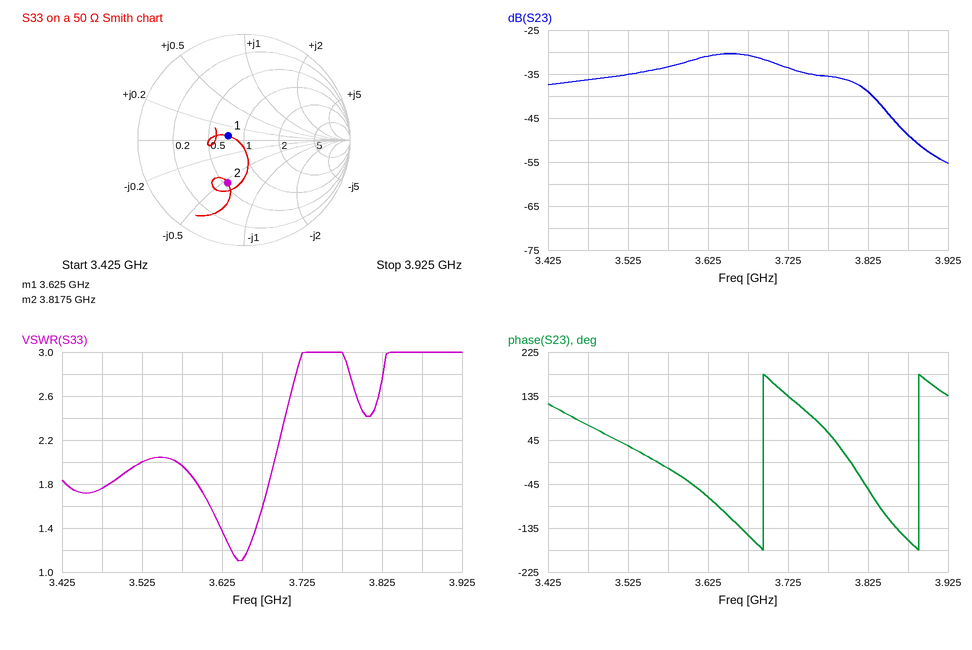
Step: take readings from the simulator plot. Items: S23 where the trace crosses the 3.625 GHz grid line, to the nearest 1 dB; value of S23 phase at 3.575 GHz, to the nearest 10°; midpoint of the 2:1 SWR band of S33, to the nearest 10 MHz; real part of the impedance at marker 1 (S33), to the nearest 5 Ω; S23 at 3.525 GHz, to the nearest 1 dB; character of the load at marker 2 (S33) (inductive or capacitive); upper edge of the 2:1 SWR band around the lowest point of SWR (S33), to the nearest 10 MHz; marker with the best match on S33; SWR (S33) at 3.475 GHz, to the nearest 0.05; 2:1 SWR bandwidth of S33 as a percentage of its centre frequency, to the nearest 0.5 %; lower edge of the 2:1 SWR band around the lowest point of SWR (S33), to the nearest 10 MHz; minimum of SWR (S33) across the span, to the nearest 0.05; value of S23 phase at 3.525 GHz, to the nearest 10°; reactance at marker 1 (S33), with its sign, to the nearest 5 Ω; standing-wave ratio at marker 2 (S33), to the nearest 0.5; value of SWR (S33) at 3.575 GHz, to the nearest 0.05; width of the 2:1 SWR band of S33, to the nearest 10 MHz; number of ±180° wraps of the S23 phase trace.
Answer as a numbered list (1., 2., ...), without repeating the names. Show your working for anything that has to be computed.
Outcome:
1. -31 dB
2. -10°
3. 3.63 GHz
4. 35 Ω
5. -35 dB
6. capacitive
7. 3.69 GHz
8. marker 1
9. 1.75
10. 120 MHz / 3.63 GHz ≈ 3.31 %, so 3.5 % to the nearest 0.5 %
11. 3.57 GHz
12. 1.10
13. 30°
14. +5 Ω
15. 2.5
16. 1.95
17. 3.69 GHz − 3.57 GHz = 120 MHz
18. 2
